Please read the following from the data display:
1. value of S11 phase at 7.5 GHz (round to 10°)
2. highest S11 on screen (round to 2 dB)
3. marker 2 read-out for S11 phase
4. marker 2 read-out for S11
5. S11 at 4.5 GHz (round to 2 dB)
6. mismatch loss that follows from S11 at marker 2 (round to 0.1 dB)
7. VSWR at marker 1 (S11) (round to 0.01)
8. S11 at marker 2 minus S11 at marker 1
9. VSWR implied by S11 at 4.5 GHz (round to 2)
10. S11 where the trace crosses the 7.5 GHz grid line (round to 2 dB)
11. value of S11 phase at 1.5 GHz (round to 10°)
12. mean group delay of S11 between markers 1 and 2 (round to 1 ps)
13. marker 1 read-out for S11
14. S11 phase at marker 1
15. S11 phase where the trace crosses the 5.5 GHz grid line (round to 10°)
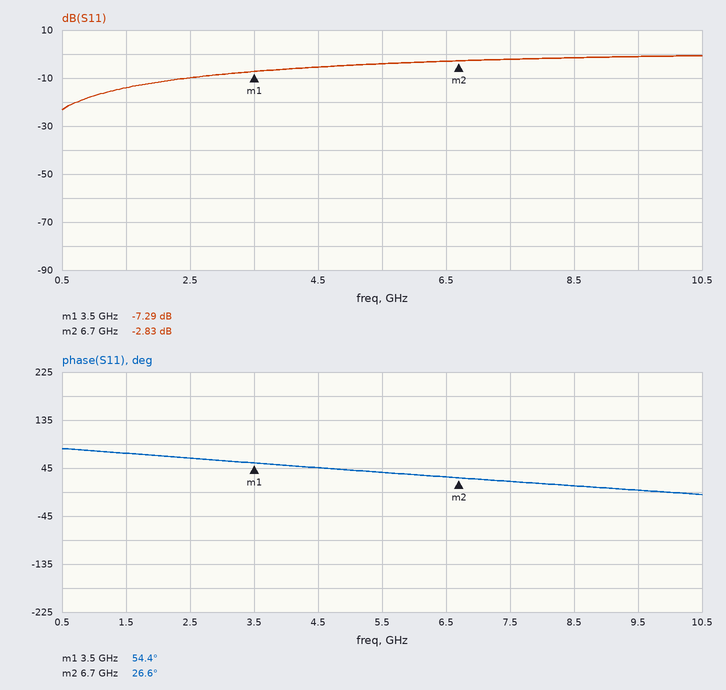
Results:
20°
0 dB
26.6°
-2.83 dB
-6 dB
3.2 dB
2.52
4.46 dB
4
-2 dB
70°
24 ps
-7.29 dB
54.4°
40°
